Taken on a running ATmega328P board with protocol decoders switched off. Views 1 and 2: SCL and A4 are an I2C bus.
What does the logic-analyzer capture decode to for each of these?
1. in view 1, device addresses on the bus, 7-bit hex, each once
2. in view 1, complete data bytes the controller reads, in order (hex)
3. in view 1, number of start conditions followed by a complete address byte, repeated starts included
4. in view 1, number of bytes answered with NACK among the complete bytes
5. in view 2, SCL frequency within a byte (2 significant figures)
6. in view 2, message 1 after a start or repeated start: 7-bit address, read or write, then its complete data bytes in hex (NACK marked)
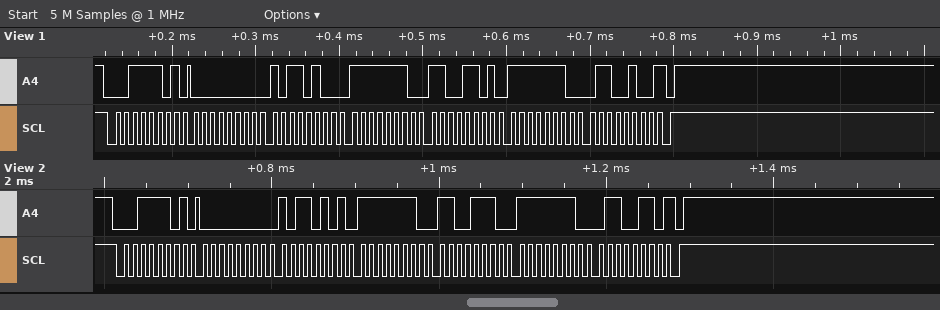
0x1E
00 B4 FE CD FE 64
1
1
100 kHz
0x1E read: 00 B5 FE CE FE 66 NACK
